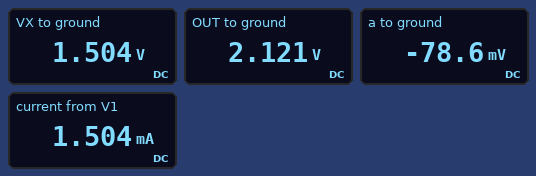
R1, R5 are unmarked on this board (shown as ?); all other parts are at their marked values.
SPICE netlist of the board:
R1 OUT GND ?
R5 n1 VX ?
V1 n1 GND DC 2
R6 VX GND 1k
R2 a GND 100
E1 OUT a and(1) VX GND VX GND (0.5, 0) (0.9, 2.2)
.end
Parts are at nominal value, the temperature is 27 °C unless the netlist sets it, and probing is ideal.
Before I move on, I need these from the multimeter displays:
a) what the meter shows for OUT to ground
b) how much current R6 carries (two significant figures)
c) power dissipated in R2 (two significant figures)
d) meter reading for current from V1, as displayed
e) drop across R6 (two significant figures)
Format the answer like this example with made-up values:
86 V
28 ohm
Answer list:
2.121 V
1.5 mA
62 µW
1.504 mA
1.5 V
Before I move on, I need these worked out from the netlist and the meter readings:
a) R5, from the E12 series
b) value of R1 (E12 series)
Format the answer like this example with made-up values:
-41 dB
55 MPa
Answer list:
330 Ω
2.7 kΩ
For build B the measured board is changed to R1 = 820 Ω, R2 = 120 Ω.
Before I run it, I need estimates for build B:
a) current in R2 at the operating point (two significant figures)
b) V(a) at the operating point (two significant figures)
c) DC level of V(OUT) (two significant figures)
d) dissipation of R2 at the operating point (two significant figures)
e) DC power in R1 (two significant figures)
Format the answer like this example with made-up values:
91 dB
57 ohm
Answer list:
2.3 mA
-280 mV
1.9 V
660 µW
4.5 mW
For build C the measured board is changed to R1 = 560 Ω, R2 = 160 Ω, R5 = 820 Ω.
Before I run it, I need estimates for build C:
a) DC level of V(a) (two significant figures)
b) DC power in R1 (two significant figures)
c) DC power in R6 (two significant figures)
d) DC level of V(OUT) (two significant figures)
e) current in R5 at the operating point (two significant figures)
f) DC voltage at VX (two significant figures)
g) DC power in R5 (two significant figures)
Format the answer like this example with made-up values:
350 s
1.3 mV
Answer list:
-490 mV
5.2 mW
1.2 mW
1.7 V
1.1 mA
1.1 V
990 µW
